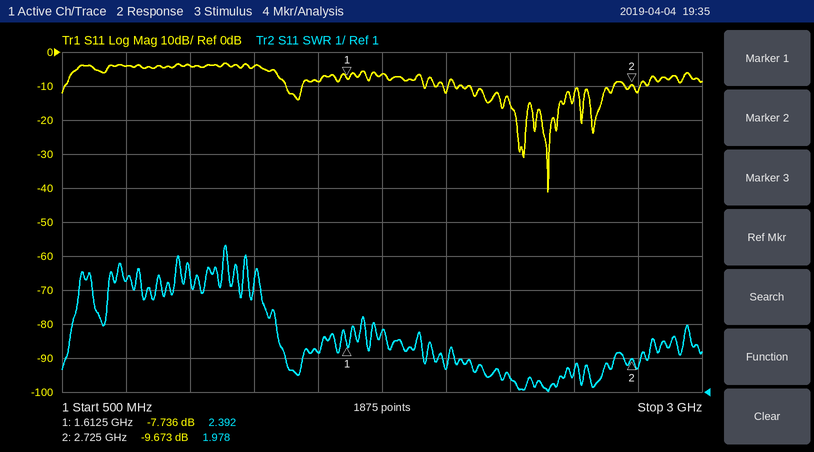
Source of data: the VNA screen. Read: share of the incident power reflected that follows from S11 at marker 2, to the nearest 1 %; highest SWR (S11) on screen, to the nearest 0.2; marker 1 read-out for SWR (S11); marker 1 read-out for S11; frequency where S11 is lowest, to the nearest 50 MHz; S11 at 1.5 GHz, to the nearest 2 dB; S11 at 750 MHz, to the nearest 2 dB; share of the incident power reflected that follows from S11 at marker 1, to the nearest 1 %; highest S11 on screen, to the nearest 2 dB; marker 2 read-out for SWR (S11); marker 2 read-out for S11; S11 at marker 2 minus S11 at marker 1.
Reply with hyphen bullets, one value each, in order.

- 11 %
- 5.4
- 2.392
- -7.736 dB
- 2.40 GHz
- -8 dB
- -4 dB
- 17 %
- -4 dB
- 1.978
- -9.673 dB
- -1.937 dB
